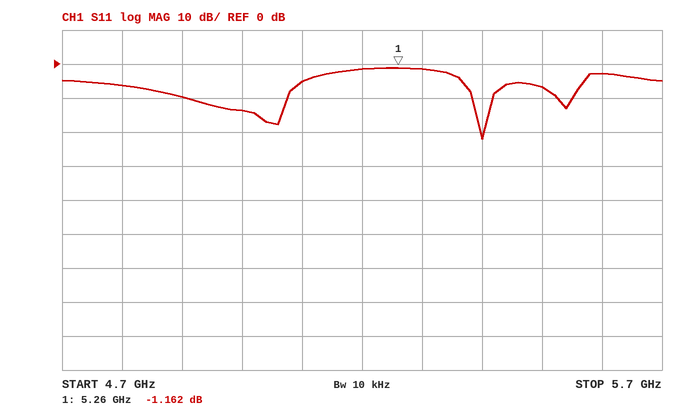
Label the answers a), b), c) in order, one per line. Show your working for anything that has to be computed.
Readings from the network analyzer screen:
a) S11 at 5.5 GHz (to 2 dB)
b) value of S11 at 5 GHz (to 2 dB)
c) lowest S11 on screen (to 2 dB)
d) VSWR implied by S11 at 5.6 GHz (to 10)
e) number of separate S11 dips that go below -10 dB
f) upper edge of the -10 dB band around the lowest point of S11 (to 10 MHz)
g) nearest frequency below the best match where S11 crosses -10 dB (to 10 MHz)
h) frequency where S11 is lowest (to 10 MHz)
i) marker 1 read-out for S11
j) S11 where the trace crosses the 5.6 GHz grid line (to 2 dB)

a) -6 dB
b) -14 dB
c) -22 dB
d) |Γ| = 10^(-2/20) = 0.7943; VSWR = (1 + 0.7943)/(1 − 0.7943) ≈ 8.72, so 10 to the nearest 10
e) 3
f) 5.42 GHz
g) 5.38 GHz
h) 5.40 GHz
i) -1.162 dB
j) -2 dB
